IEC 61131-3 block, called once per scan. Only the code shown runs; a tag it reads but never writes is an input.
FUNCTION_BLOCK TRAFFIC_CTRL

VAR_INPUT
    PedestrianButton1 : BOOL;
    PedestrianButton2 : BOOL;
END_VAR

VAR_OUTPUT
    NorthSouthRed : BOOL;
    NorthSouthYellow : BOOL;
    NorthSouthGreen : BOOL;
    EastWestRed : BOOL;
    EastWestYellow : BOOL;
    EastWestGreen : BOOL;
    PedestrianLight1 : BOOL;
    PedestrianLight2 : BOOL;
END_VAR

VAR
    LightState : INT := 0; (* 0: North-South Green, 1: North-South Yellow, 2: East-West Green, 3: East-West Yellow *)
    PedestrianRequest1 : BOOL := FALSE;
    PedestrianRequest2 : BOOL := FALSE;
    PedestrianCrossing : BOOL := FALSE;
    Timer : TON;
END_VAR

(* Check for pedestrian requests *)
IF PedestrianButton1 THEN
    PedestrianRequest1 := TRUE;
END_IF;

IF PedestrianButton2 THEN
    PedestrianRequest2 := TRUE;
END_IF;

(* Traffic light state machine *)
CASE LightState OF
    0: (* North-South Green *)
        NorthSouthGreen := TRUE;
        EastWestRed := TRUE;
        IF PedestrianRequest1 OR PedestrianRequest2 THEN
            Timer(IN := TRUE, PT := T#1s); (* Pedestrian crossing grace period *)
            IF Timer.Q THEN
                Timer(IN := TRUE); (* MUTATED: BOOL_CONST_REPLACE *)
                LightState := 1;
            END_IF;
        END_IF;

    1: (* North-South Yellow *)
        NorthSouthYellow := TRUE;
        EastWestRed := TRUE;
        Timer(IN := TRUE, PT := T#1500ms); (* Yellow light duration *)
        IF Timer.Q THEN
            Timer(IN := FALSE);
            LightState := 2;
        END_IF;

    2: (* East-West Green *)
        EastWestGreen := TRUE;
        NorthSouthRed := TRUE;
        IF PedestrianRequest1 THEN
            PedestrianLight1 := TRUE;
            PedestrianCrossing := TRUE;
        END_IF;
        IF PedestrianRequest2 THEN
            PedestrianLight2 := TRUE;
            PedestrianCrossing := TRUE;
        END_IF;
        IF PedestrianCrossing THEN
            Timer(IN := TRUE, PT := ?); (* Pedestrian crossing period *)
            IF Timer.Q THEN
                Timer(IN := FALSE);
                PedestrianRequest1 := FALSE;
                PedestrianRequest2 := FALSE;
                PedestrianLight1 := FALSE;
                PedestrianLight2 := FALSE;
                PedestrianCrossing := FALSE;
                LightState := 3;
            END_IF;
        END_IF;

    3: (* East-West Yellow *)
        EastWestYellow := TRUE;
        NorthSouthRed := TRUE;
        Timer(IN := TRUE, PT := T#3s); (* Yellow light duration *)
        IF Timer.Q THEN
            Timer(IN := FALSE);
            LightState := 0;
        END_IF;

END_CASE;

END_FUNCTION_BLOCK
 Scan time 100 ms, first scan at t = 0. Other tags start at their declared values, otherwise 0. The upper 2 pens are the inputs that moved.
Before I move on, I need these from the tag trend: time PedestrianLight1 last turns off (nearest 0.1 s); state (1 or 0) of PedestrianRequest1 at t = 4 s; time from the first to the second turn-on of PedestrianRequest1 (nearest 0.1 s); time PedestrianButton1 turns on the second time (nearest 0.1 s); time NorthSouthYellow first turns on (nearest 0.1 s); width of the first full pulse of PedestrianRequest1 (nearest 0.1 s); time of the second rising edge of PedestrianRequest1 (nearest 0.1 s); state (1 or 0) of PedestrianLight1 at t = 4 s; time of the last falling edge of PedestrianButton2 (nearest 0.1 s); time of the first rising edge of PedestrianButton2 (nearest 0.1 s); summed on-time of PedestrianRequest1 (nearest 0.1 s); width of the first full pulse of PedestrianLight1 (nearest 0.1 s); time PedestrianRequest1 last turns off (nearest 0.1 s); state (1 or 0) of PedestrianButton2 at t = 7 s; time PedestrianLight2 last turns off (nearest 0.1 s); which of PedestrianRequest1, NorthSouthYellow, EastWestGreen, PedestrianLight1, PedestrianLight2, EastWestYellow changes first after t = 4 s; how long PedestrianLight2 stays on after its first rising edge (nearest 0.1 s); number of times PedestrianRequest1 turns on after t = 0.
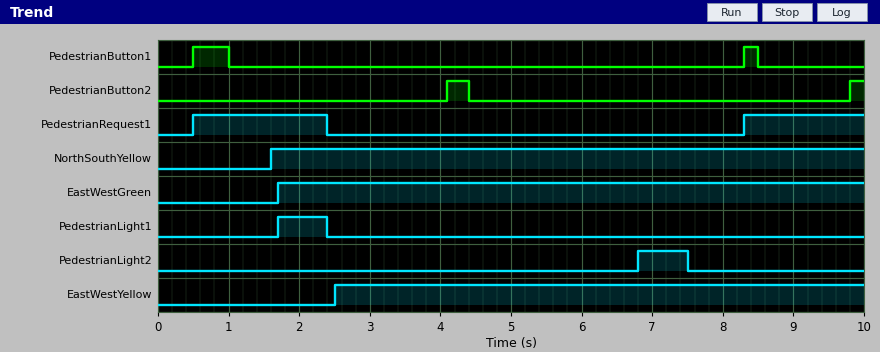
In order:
2.4 s
0
7.8 s
8.3 s
1.6 s
1.9 s
8.3 s
0
4.4 s
4.1 s
3.6 s
0.7 s
2.4 s
0
7.5 s
PedestrianLight2
0.7 s
2
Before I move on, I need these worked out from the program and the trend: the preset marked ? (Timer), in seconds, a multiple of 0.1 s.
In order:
0.7 s
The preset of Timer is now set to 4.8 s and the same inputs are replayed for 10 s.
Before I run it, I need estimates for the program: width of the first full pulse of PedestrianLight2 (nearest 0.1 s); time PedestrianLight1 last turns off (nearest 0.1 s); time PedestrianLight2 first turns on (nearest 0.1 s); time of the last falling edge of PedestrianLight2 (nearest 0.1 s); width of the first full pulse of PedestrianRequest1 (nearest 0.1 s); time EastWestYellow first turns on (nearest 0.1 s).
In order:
2.4 s
6.5 s
4.1 s
6.5 s
6.0 s
6.6 s
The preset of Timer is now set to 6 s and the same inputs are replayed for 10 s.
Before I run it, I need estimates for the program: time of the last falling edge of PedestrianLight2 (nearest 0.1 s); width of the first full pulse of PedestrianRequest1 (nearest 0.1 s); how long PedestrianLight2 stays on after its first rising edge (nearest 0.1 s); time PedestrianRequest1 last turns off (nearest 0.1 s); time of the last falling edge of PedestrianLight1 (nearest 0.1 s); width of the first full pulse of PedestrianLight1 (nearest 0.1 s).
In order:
7.7 s
7.2 s
3.6 s
7.7 s
7.7 s
6.0 s
